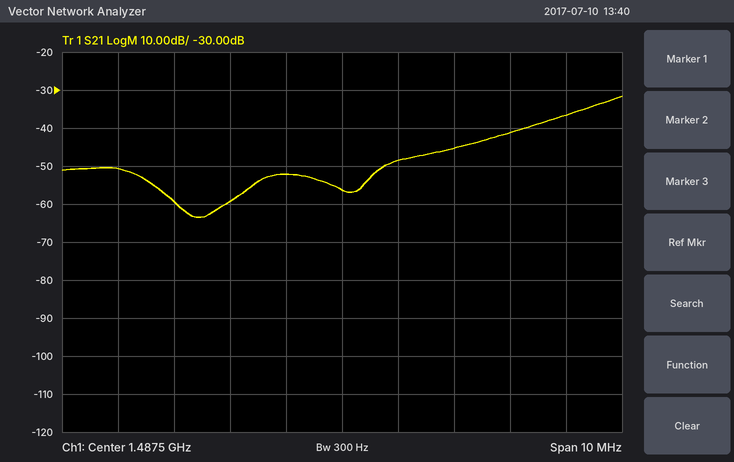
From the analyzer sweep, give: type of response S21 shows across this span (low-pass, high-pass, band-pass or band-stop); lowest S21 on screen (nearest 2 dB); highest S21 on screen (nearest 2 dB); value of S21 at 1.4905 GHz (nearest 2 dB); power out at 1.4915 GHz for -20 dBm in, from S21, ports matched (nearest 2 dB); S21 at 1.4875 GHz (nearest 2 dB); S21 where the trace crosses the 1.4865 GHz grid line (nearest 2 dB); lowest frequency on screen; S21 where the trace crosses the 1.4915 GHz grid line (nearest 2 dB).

high-pass
-64 dB
-32 dB
-42 dB
-56 dBm
-56 dB
-52 dB
1.4825 GHz
-36 dB
